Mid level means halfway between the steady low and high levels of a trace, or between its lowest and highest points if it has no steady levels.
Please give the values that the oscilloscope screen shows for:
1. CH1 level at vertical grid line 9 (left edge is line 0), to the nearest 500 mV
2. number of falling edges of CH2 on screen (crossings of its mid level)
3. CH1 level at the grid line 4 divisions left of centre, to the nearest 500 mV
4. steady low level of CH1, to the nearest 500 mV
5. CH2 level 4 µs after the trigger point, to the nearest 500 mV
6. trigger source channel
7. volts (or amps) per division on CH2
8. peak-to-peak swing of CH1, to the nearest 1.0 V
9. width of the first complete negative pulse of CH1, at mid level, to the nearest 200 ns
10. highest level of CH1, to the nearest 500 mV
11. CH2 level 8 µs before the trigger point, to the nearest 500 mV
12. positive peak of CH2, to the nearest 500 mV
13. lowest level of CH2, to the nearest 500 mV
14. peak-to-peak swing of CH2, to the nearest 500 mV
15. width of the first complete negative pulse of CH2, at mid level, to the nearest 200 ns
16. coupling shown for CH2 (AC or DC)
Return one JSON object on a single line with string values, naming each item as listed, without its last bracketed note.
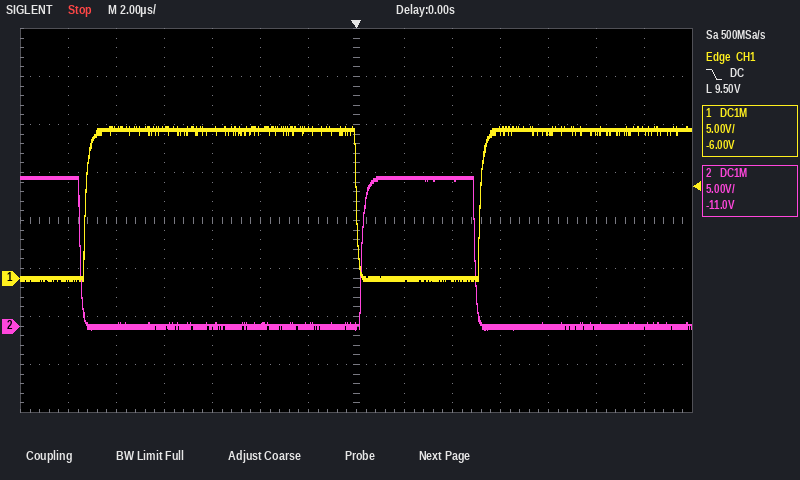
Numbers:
{"CH1 level at vertical grid line 9 (left edge is line 0), to the nearest 500 mV": "0.0 V", "number of falling edges of CH2 on screen": "2", "CH1 level at the grid line 4 divisions left of centre, to the nearest 500 mV": "15.5 V", "steady low level of CH1, to the nearest 500 mV": "0.0 V", "CH2 level 4 µs after the trigger point, to the nearest 500 mV": "15.5 V", "trigger source channel": "CH1", "volts (or amps) per division on CH2": "5 V", "peak-to-peak swing of CH1, to the nearest 1.0 V": "16.0 V", "width of the first complete negative pulse of CH1, at mid level, to the nearest 200 ns": "5.2 µs", "highest level of CH1, to the nearest 500 mV": "16.0 V", "CH2 level 8 µs before the trigger point, to the nearest 500 mV": "0.0 V", "positive peak of CH2, to the nearest 500 mV": "15.5 V", "lowest level of CH2, to the nearest 500 mV": "-500 mV", "peak-to-peak swing of CH2, to the nearest 500 mV": "16.0 V", "width of the first complete negative pulse of CH2, at mid level, to the nearest 200 ns": "11.8 µs", "coupling shown for CH2": "DC"}
